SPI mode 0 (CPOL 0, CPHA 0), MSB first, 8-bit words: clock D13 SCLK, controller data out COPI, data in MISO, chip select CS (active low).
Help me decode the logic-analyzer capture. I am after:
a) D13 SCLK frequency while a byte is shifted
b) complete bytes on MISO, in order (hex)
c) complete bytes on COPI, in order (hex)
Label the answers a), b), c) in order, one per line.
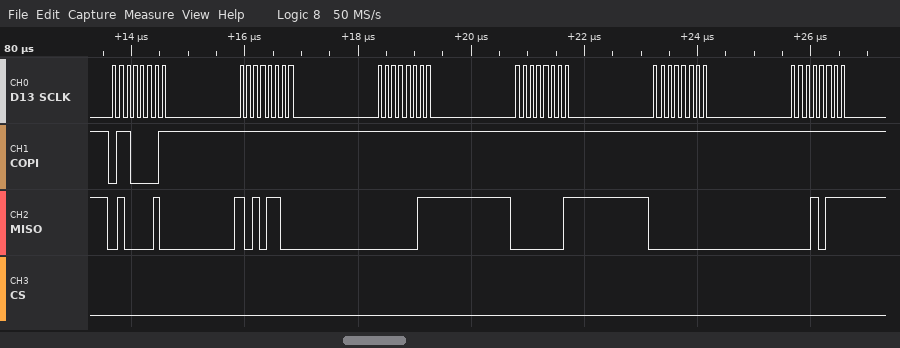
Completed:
a) 8 MHz
b) 42 AC 03 01 00 17
c) 61 FF FF FF FF FF
